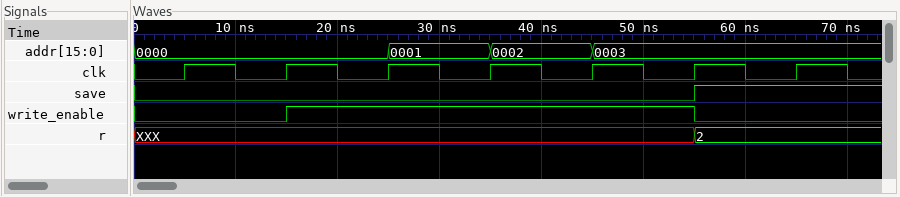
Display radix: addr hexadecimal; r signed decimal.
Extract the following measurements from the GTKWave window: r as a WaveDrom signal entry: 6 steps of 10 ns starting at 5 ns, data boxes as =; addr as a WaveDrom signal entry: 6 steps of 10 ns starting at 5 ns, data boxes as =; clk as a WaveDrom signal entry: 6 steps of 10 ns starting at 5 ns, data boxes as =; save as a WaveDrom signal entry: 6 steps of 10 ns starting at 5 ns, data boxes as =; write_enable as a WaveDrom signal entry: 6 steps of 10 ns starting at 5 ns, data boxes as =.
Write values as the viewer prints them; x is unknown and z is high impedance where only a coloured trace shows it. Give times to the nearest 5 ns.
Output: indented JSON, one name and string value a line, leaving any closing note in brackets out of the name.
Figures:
{
  "r as a WaveDrom signal entry: 6 steps of 10 ns starting at 5 ns, data boxes as =": "{name: 'r', wave: 'x....=', data: '2'}",
  "addr as a WaveDrom signal entry: 6 steps of 10 ns starting at 5 ns, data boxes as =": "{name: 'addr', wave: '=.===.', data: '0000 0001 0002 0003'}",
  "clk as a WaveDrom signal entry: 6 steps of 10 ns starting at 5 ns, data boxes as =": "{name: 'clk', wave: 'p.....'}",
  "save as a WaveDrom signal entry: 6 steps of 10 ns starting at 5 ns, data boxes as =": "{name: 'save', wave: '0....1'}",
  "write_enable as a WaveDrom signal entry: 6 steps of 10 ns starting at 5 ns, data boxes as =": "{name: 'write_enable', wave: '01...0'}"
}
